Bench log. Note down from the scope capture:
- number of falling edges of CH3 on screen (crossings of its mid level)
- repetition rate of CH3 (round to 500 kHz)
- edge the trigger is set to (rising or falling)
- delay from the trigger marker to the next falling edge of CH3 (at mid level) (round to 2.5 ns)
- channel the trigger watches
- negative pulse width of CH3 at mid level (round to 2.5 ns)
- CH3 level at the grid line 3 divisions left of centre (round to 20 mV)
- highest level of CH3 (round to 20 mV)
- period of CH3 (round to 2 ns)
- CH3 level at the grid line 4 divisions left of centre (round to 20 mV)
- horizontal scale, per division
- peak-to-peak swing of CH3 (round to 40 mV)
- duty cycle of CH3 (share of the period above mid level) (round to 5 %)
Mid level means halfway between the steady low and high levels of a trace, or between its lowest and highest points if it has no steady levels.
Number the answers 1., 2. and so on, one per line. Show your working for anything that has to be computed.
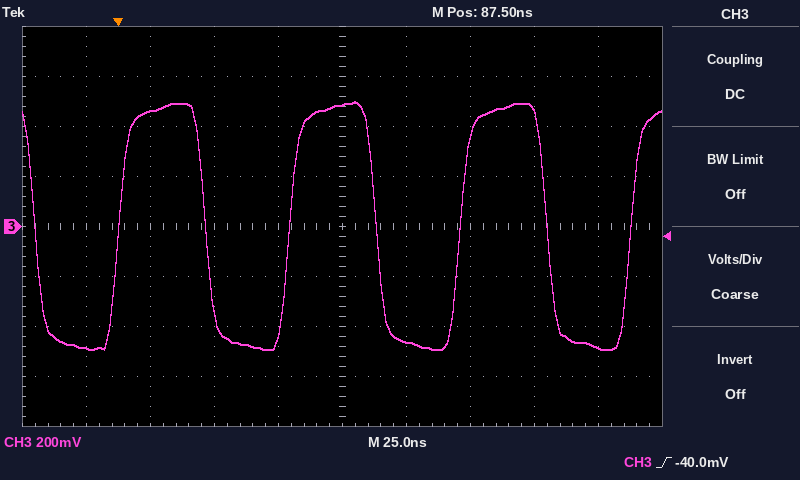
1. 4
2. 1 / 66 ns ≈ 15.2 MHz, so 15.0 MHz to the nearest 500 kHz
3. rising
4. 35.0 ns
5. CH3
6. 32.5 ns
7. 460 mV
8. 500 mV
9. 66 ns
10. -480 mV
11. 25 ns
12. 1.00 V
13. 50 %
